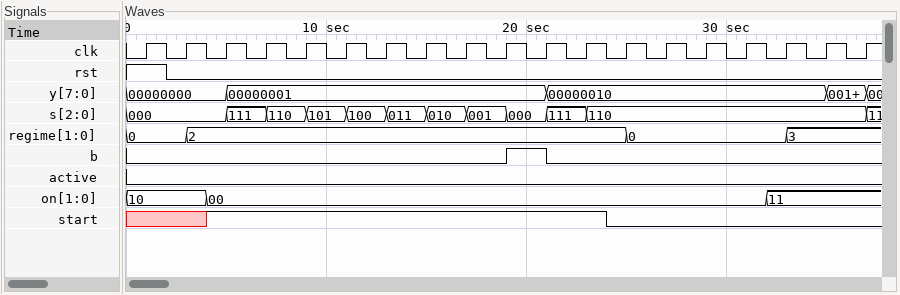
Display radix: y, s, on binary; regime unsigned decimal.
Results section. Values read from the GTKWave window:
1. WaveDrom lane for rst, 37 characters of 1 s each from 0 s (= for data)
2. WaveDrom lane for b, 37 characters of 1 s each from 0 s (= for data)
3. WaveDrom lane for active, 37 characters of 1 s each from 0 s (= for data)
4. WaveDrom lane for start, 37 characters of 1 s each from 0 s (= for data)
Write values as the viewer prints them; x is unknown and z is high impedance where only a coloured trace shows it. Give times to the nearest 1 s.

{name: 'rst', wave: '1.0..................................'}
{name: 'b', wave: '0..................1.0...............'}
{name: 'active', wave: '0....................................'}
{name: 'start', wave: 'x...1...................0............'}
